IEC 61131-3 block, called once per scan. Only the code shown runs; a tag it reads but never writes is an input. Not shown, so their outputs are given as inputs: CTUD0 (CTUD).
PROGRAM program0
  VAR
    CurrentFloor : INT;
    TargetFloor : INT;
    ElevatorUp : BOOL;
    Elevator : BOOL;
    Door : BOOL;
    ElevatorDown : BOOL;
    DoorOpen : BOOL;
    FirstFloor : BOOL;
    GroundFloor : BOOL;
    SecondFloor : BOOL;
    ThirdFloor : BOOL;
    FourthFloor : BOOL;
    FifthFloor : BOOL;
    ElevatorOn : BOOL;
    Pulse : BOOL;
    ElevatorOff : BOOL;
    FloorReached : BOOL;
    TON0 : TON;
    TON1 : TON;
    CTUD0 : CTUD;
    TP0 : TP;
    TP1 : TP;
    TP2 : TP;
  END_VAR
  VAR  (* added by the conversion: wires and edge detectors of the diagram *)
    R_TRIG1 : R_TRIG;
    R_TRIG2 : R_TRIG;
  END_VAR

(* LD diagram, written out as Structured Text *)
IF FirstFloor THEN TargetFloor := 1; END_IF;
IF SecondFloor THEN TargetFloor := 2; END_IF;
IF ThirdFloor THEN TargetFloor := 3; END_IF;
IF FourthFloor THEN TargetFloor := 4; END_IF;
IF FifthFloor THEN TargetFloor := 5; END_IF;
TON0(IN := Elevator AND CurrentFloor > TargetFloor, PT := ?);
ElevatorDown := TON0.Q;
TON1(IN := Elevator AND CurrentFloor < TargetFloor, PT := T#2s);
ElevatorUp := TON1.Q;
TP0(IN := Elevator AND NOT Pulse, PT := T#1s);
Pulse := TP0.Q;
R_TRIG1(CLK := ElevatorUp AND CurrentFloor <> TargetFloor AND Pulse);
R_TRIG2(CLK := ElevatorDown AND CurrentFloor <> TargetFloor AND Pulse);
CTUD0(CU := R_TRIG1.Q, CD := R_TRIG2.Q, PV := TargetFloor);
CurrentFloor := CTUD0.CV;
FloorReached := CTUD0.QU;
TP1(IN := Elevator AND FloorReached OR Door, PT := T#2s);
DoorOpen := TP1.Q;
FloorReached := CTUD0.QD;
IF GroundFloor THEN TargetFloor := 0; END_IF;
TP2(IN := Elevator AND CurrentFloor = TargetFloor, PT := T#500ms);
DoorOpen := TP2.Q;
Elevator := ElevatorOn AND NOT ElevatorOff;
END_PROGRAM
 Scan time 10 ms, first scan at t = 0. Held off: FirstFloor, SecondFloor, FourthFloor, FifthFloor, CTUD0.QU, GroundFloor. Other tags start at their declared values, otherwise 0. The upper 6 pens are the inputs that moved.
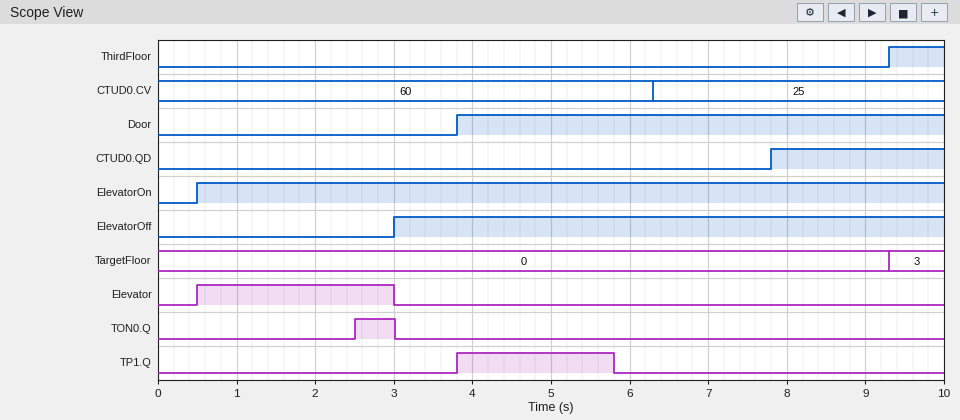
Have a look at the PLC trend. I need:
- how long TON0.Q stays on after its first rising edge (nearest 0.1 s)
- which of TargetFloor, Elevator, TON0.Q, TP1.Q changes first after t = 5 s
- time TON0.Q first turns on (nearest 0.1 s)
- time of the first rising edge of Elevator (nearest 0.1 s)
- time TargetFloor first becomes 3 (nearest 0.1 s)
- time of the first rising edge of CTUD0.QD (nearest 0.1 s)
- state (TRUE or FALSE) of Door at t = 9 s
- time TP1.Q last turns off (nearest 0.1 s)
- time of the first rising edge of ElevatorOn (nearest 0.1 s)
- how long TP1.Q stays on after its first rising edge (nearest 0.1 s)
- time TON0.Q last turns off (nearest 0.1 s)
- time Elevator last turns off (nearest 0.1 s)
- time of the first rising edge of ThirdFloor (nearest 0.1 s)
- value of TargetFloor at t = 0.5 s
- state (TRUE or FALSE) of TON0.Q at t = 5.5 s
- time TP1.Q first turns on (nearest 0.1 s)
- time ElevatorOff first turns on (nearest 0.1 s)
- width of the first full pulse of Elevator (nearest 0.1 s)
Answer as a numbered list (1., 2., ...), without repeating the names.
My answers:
1. 0.5 s
2. TP1.Q
3. 2.5 s
4. 0.5 s
5. 9.3 s
6. 7.8 s
7. TRUE
8. 5.8 s
9. 0.5 s
10. 2.0 s
11. 3.0 s
12. 3.0 s
13. 9.3 s
14. 0
15. FALSE
16. 3.8 s
17. 3.0 s
18. 2.5 s
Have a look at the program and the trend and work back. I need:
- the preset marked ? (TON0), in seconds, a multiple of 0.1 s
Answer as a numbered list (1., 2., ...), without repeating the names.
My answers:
1. 2.0 s
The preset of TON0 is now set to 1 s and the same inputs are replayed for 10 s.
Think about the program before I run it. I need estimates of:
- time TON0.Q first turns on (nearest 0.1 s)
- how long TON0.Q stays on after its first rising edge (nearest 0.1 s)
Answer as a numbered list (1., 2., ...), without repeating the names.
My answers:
1. 1.5 s
2. 1.5 s
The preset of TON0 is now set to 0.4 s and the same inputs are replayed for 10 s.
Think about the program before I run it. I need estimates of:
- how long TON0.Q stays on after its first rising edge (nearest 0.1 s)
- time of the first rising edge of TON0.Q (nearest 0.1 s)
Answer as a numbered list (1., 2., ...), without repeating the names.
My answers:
1. 2.1 s
2. 0.9 s
